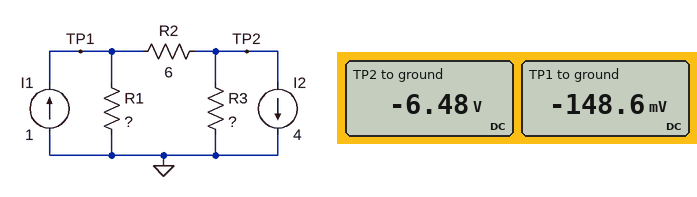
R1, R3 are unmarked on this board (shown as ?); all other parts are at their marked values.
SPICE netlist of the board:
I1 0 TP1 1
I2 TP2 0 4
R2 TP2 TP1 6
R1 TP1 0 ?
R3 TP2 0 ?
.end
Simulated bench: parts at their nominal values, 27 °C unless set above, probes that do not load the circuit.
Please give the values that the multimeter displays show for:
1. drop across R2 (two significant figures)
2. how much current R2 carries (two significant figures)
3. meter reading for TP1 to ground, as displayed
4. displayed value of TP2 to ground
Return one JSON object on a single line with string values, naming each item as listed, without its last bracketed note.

{"drop across R2": "6.3 V", "how much current R2 carries": "1.1 A", "meter reading for TP1 to ground, as displayed": "-148.6 mV", "displayed value of TP2 to ground": "-6.48 V"}
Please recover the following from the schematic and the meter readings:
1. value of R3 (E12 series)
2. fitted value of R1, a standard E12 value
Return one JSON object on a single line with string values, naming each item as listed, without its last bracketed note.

{"value of R3": "2.2 Ω", "fitted value of R1, a standard E12 value": "2.7 Ω"}
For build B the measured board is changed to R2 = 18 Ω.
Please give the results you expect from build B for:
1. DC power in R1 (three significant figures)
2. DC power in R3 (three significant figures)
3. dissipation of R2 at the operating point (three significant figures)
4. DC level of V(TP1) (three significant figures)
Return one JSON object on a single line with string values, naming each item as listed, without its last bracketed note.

{"DC power in R1": "669 mW", "DC power in R3": "26.9 W", "dissipation of R2 at the operating point": "4.54 W", "DC level of V(TP1)": "1.34 V"}
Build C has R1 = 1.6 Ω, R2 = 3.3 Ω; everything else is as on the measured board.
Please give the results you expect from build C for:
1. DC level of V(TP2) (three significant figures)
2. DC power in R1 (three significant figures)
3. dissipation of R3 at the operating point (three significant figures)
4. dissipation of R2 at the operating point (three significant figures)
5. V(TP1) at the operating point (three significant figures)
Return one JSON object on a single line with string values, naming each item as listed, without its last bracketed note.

{"DC level of V(TP2)": "-5.58 V", "DC power in R1": "346 mW", "dissipation of R3 at the operating point": "14.1 W", "dissipation of R2 at the operating point": "7.08 W", "V(TP1) at the operating point": "-744 mV"}
